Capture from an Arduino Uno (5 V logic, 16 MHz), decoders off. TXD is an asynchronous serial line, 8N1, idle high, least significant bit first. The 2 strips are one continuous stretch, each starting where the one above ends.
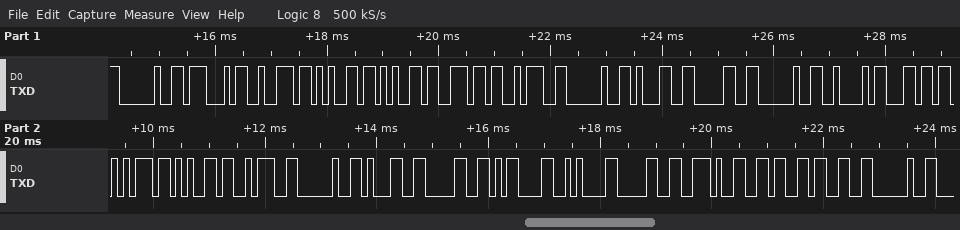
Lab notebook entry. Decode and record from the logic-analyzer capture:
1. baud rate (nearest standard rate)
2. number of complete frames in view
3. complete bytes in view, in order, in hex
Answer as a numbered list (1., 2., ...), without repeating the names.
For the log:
1. 9600 baud
2. 26
3. 0x20 0x47 0x72 0x65 0x65 0x6E 0x3A 0x20 0x31 0x30 0x20 0x42 0x6C 0x75 0x65 0x3A 0x20 0x31 0x30 0x0D 0x0A 0x30 0x2E 0x36 0x33 0x20
